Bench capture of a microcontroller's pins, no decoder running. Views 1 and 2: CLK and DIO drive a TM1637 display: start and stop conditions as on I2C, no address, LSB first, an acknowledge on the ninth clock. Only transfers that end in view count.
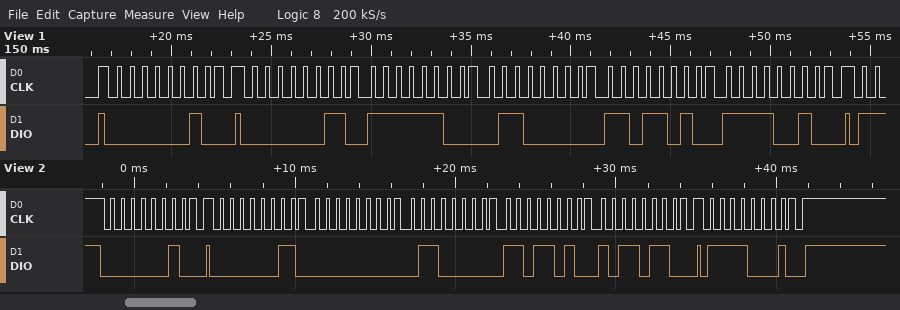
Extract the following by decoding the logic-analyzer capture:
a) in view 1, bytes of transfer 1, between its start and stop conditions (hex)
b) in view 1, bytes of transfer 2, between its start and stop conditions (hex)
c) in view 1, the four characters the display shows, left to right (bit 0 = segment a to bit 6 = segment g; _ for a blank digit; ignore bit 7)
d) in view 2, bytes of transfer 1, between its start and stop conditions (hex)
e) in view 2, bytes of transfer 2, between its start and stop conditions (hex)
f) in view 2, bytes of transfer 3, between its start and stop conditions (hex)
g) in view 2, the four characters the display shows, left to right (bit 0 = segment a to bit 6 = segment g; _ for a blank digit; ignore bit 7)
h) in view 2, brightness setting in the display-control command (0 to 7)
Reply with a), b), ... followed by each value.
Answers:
a) 40
b) C0 3F 06 5B 4F
c) 0123
d) 40
e) C0 00 06 5B 6D
f) 8F
g) _125
h) 7
